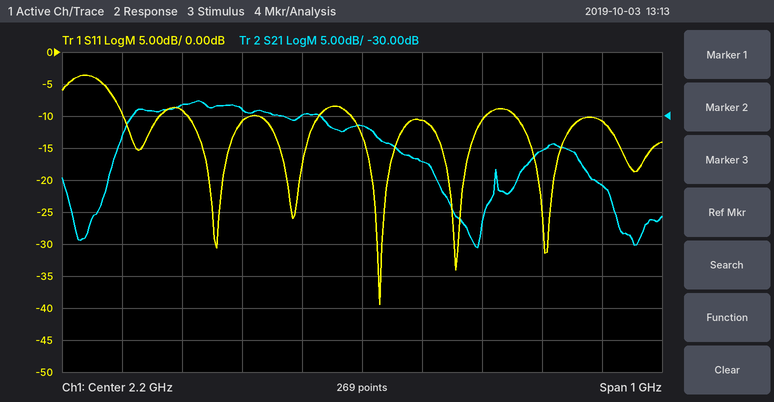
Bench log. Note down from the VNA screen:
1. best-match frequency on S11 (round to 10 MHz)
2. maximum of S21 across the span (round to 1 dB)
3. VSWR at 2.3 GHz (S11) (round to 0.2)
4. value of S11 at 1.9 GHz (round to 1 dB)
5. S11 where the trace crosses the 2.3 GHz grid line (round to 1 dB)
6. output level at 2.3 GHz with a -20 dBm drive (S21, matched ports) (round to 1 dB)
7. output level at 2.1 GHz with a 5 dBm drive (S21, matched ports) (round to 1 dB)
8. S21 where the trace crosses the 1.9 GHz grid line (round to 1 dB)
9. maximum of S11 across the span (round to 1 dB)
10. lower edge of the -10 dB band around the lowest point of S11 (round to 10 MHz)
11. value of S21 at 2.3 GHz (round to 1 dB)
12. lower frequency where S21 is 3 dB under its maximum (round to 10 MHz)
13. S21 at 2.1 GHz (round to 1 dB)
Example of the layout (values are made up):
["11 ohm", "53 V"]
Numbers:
["2.23 GHz", "-28 dB", "1.8", "-9 dB", "-11 dB", "-57 dBm", "-25 dBm", "-28 dB", "-4 dB", "2.18 GHz", "-37 dB", "1.81 GHz", "-30 dB"]
